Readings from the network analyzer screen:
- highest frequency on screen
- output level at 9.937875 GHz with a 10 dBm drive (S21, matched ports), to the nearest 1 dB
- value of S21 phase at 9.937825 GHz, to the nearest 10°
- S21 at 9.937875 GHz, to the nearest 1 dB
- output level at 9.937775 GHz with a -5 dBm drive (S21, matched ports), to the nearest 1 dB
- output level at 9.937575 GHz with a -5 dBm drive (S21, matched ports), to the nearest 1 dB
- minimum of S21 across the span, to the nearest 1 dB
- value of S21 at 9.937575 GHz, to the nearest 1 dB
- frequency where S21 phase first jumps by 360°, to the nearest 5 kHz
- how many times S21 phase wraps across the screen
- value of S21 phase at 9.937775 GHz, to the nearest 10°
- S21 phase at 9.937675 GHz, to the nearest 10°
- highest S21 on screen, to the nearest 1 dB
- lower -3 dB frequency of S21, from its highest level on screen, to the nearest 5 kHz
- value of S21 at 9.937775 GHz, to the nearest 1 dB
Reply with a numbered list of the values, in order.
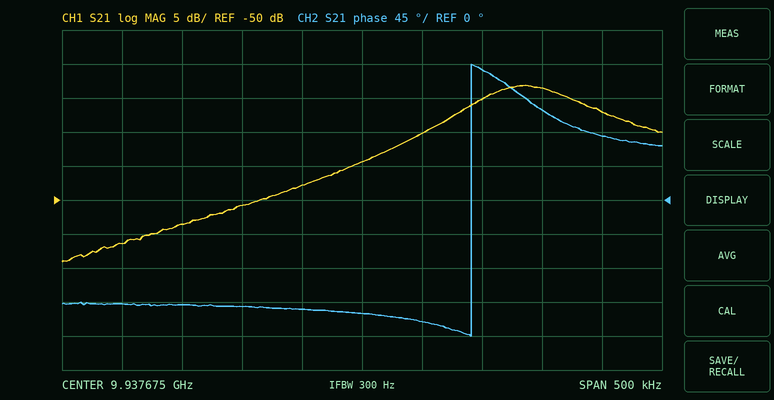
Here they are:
1. 9.937925 GHz
2. -27 dBm
3. 120°
4. -37 dB
5. -40 dBm
6. -56 dBm
7. -59 dB
8. -51 dB
9. 9.937765 GHz
10. 1
11. 170°
12. -150°
13. -33 dB
14. 9.937765 GHz
15. -35 dB
